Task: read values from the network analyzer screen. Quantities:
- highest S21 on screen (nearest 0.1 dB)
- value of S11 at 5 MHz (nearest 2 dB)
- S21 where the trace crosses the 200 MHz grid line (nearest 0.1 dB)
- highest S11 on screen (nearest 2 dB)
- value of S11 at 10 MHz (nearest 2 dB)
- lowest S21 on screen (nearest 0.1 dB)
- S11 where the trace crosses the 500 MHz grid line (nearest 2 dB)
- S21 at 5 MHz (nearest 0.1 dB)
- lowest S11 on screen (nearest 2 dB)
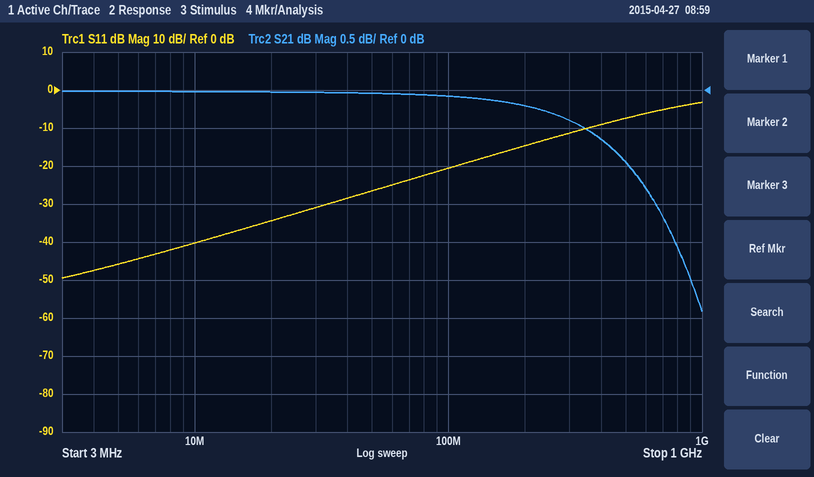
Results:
0.0 dB
-46 dB
-0.2 dB
-4 dB
-40 dB
-2.9 dB
-8 dB
0.0 dB
-50 dB
